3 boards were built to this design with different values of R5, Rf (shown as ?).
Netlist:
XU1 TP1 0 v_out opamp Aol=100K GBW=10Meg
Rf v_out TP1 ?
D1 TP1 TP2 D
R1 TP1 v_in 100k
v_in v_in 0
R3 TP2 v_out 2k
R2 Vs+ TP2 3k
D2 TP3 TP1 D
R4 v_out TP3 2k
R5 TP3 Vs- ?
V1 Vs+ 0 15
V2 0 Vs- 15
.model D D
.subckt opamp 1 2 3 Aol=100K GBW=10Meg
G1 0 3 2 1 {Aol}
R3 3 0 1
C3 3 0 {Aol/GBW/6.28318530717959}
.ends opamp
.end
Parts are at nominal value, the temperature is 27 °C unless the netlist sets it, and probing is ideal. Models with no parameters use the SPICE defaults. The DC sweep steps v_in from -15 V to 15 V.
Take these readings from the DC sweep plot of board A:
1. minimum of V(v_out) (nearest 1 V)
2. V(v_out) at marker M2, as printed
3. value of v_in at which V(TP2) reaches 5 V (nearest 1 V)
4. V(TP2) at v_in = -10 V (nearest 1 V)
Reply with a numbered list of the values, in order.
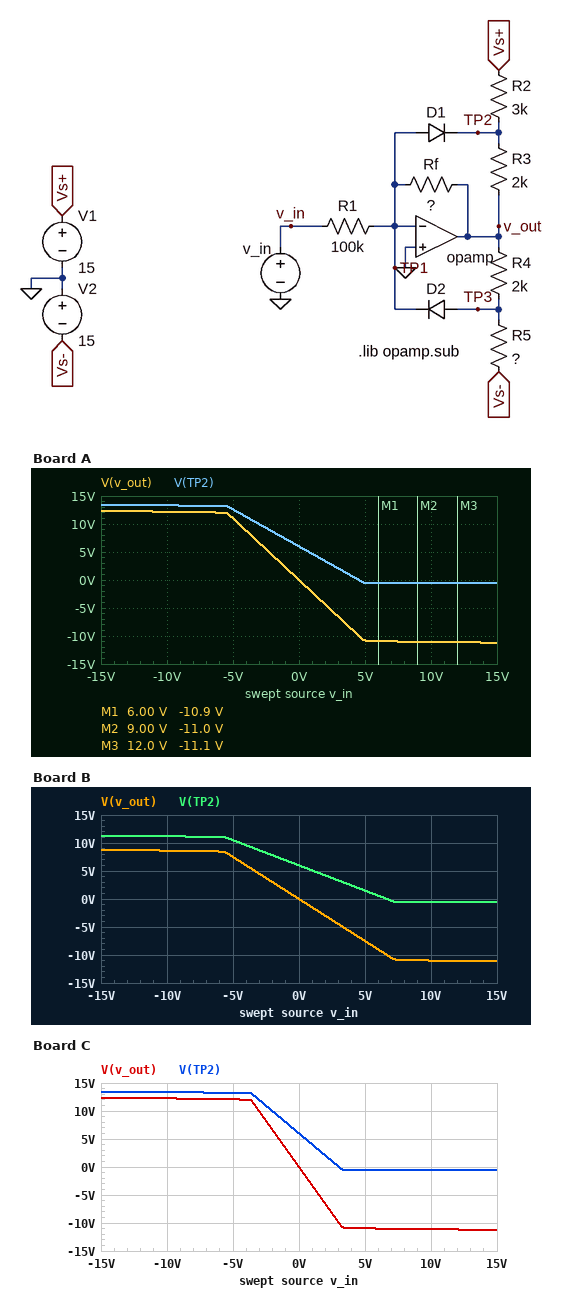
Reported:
1. -11 V
2. -11.0 V
3. 1 V
4. 13 V
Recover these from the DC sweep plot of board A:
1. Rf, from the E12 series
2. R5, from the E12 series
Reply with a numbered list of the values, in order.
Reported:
1. 220 kΩ
2. 2.7 kΩ
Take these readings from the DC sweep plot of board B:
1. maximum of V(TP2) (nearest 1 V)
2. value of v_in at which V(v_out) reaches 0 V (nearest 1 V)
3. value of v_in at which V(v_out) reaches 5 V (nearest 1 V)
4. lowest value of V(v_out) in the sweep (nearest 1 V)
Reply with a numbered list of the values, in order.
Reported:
1. 11 V
2. 0 V
3. -3 V
4. -11 V
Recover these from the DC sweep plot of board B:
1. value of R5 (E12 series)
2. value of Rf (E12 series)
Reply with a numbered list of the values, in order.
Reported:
1. 3.9 kΩ
2. 150 kΩ
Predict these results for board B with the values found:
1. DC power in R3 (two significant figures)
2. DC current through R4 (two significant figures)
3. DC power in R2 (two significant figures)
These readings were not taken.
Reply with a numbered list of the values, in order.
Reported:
1. 18 mW
2. 2.5 mA
3. 27 mW
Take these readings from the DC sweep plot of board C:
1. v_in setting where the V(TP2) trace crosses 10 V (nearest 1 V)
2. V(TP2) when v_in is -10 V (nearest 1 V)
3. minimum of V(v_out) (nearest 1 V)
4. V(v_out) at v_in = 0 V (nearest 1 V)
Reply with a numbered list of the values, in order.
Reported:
1. -2 V
2. 13 V
3. -11 V
4. 0 V
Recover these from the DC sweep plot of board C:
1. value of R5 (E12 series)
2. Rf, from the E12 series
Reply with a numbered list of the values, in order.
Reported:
1. 2.7 kΩ
2. 330 kΩ
